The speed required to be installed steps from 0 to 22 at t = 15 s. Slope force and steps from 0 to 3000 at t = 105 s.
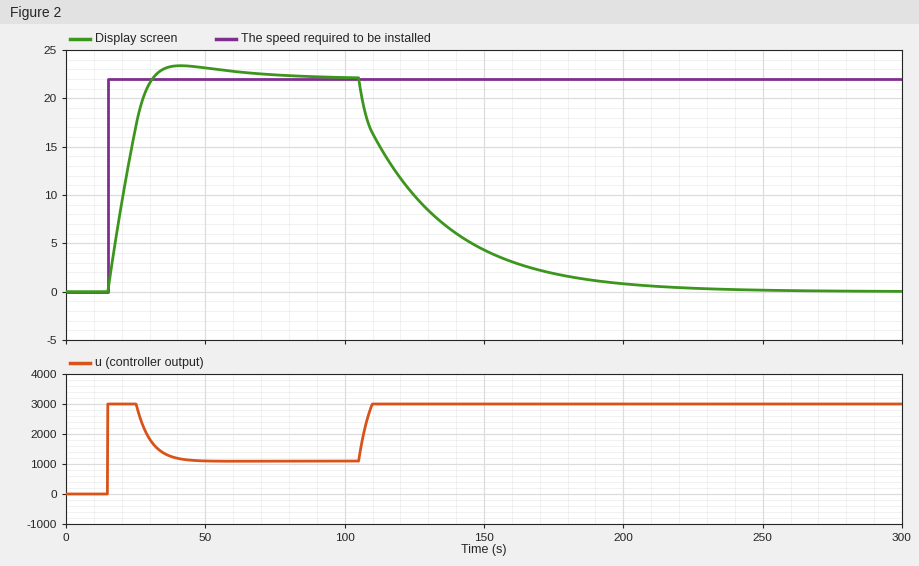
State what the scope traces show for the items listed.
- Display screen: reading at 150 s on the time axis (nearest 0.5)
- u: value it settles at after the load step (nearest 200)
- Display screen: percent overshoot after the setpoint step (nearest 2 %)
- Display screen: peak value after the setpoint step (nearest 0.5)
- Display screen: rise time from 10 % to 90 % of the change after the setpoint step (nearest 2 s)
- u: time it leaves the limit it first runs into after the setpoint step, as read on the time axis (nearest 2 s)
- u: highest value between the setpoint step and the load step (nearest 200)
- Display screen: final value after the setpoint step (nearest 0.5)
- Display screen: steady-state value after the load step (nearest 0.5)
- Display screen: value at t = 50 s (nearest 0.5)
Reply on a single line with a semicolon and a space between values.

4.5; 3000; 6 %; 23.5; 12 s; 26 s; 3000; 22.0; 0.0; 23.0
